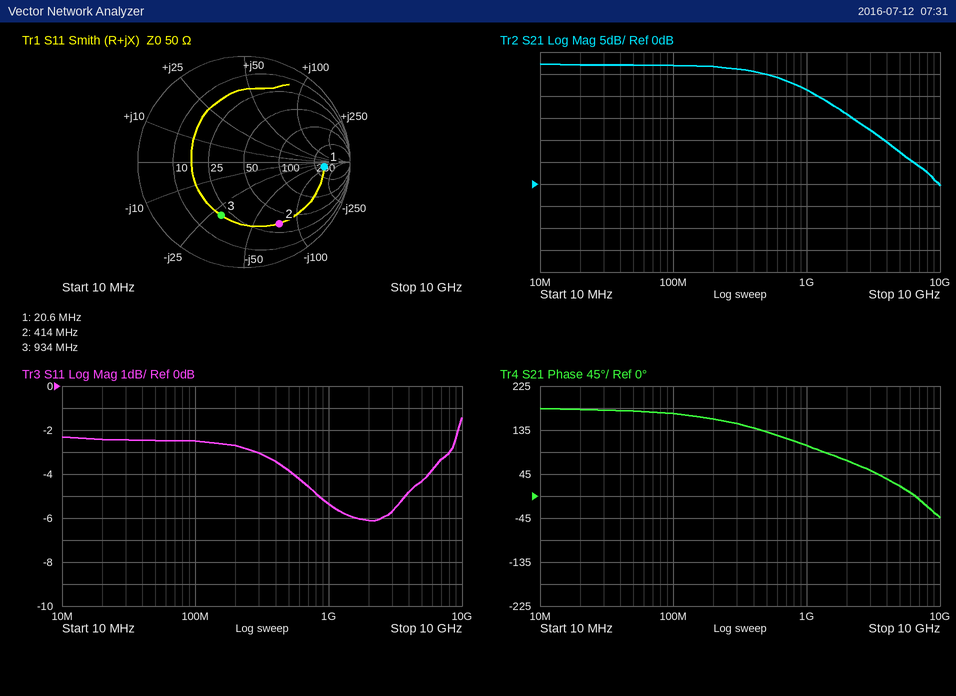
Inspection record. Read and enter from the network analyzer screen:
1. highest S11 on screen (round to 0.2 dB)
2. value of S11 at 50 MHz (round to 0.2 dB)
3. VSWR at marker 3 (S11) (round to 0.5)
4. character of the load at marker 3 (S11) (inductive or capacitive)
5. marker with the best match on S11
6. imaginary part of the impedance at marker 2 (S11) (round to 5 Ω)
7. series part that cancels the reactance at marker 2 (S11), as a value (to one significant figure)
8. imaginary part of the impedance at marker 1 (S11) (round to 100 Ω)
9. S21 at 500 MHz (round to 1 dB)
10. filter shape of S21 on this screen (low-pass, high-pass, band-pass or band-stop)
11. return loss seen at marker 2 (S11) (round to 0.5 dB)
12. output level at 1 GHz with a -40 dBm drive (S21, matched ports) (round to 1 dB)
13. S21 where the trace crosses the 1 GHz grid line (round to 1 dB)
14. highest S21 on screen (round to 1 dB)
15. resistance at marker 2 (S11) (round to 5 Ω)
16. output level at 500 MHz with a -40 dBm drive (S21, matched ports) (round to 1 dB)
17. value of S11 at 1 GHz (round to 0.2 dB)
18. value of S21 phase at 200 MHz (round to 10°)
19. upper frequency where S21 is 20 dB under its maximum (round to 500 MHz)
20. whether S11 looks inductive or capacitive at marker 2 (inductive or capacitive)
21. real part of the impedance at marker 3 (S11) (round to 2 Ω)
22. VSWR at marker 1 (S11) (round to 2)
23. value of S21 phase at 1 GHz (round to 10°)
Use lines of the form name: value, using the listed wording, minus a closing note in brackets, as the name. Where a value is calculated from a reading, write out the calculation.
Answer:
highest S11 on screen: -1.4 dB
value of S11 at 50 MHz: -2.4 dB
VSWR at marker 3 (S11): 3.5
character of the load at marker 3 (S11): capacitive
marker with the best match on S11: marker 3
imaginary part of the impedance at marker 2 (S11): -75 Ω
series part that cancels the reactance at marker 2 (S11), as a value: L = 75 Ω/(2π × 414 MHz) ≈ 28.8 nH, so 30 nH to one significant figure
imaginary part of the impedance at marker 1 (S11): -100 Ω
S21 at 500 MHz: 25 dB
filter shape of S21 on this screen: low-pass
return loss seen at marker 2 (S11): 3.5 dB
output level at 1 GHz with a -40 dBm drive (S21, matched ports): -40 dBm + (21 dB) = -19 dBm
S21 where the trace crosses the 1 GHz grid line: 21 dB
highest S21 on screen: 27 dB
resistance at marker 2 (S11): 35 Ω
output level at 500 MHz with a -40 dBm drive (S21, matched ports): -40 dBm + (25 dB) = -15 dBm
value of S11 at 1 GHz: -5.4 dB
value of S21 phase at 200 MHz: 160°
upper frequency where S21 is 20 dB under its maximum: 5.0 GHz
whether S11 looks inductive or capacitive at marker 2: capacitive
real part of the impedance at marker 3 (S11): 20 Ω
VSWR at marker 1 (S11): 8
value of S21 phase at 1 GHz: 100°
